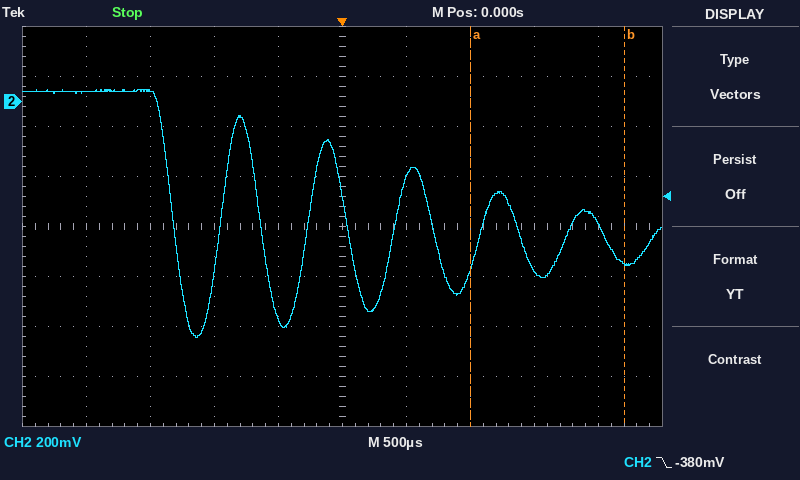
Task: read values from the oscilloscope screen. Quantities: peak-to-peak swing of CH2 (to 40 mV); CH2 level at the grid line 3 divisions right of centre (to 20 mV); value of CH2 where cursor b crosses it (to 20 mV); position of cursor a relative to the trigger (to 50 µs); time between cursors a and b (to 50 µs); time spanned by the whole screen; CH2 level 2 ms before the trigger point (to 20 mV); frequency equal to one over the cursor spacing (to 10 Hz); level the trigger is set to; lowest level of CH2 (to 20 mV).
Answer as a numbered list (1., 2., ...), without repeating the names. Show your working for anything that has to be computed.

1. 1.00 V
2. -680 mV
3. -640 mV
4. +1.00 ms
5. 1.20 ms
6. 5 ms
7. 40 mV
8. 1 / 1.20 ms ≈ 830 Hz
9. -380 mV
10. -940 mV
